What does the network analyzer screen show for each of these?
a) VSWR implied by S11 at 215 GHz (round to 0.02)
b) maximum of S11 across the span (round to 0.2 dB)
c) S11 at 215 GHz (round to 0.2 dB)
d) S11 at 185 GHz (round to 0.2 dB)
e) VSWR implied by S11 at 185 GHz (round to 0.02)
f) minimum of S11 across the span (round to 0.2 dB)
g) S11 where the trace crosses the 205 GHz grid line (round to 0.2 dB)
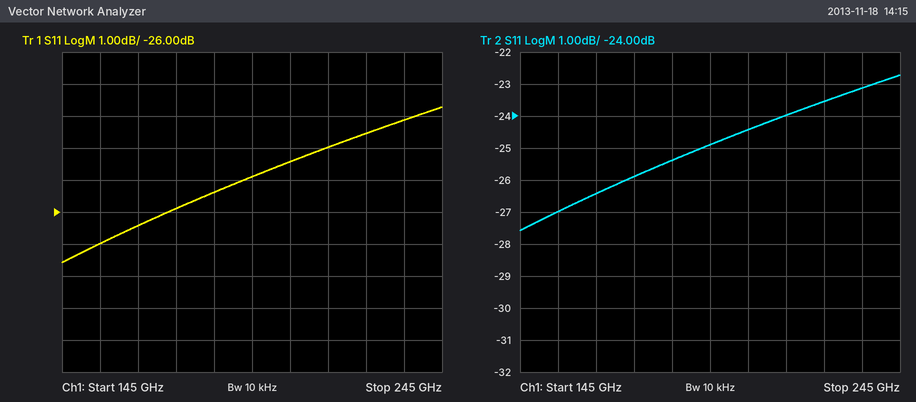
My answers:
1.14
-22.8 dB
-24.0 dB
-25.4 dB
1.12
-27.6 dB
-24.4 dB
